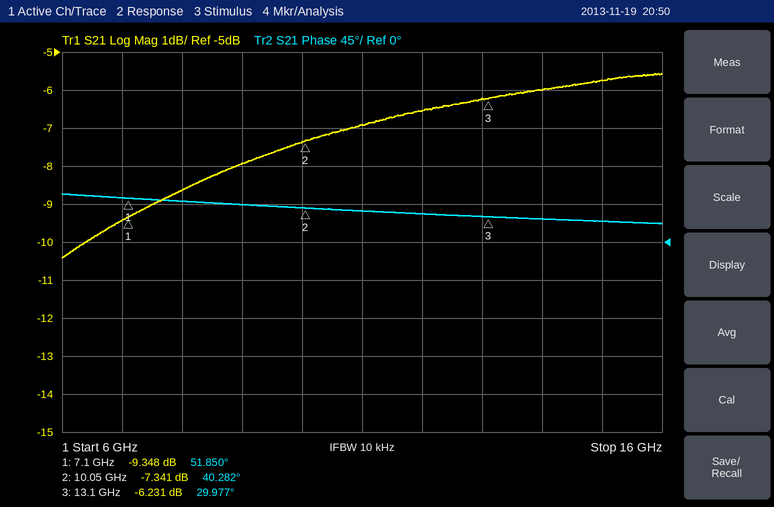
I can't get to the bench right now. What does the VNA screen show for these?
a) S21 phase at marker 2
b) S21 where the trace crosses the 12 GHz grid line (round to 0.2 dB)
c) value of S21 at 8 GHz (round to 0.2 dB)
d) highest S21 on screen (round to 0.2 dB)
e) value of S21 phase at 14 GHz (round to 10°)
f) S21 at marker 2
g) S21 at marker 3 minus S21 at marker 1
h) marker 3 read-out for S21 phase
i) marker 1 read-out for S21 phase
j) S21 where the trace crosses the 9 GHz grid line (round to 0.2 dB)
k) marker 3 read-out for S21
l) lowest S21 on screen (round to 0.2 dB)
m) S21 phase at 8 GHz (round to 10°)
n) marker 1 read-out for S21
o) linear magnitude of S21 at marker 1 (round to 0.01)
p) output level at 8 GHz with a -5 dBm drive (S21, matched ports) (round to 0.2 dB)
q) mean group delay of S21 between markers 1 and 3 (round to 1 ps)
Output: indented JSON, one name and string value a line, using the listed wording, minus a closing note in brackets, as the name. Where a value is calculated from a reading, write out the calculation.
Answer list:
{
  "S21 phase at marker 2": "40.282°",
  "S21 where the trace crosses the 12 GHz grid line": "-6.6 dB",
  "value of S21 at 8 GHz": "-8.6 dB",
  "highest S21 on screen": "-5.6 dB",
  "value of S21 phase at 14 GHz": "30°",
  "S21 at marker 2": "-7.341 dB",
  "S21 at marker 3 minus S21 at marker 1": "-6.231 − (-9.348) = 3.117 dB",
  "marker 3 read-out for S21 phase": "29.977°",
  "marker 1 read-out for S21 phase": "51.850°",
  "S21 where the trace crosses the 9 GHz grid line": "-8.0 dB",
  "marker 3 read-out for S21": "-6.231 dB",
  "lowest S21 on screen": "-10.4 dB",
  "S21 phase at 8 GHz": "50°",
  "marker 1 read-out for S21": "-9.348 dB",
  "linear magnitude of S21 at marker 1": "10^(-9.348/20) ≈ 0.34",
  "output level at 8 GHz with a -5 dBm drive (S21, matched ports)": "-5 dBm + (-8.6 dB) = -13.6 dBm",
  "mean group delay of S21 between markers 1 and 3": "−(29.977° − (51.85°))/(360° × 6 GHz) ≈ 10 ps"
}
